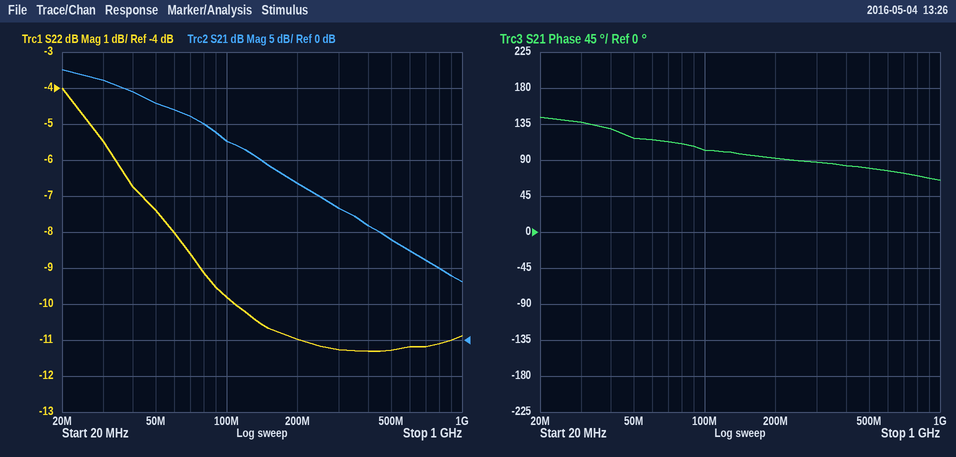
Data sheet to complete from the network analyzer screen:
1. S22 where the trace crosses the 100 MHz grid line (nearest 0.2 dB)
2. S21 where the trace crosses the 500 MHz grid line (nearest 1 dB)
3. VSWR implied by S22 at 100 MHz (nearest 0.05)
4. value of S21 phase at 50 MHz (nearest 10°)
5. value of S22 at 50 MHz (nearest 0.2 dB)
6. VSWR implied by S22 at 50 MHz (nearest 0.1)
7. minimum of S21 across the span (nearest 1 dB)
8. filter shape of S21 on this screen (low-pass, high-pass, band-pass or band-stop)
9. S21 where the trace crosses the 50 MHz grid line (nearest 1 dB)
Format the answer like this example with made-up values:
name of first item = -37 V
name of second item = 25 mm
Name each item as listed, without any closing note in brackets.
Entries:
S22 where the trace crosses the 100 MHz grid line = -9.8 dB
S21 where the trace crosses the 500 MHz grid line = 14 dB
VSWR implied by S22 at 100 MHz = 1.95
value of S21 phase at 50 MHz = 120°
value of S22 at 50 MHz = -7.4 dB
VSWR implied by S22 at 50 MHz = 2.5
minimum of S21 across the span = 8 dB
filter shape of S21 on this screen = low-pass
S21 where the trace crosses the 50 MHz grid line = 33 dB
